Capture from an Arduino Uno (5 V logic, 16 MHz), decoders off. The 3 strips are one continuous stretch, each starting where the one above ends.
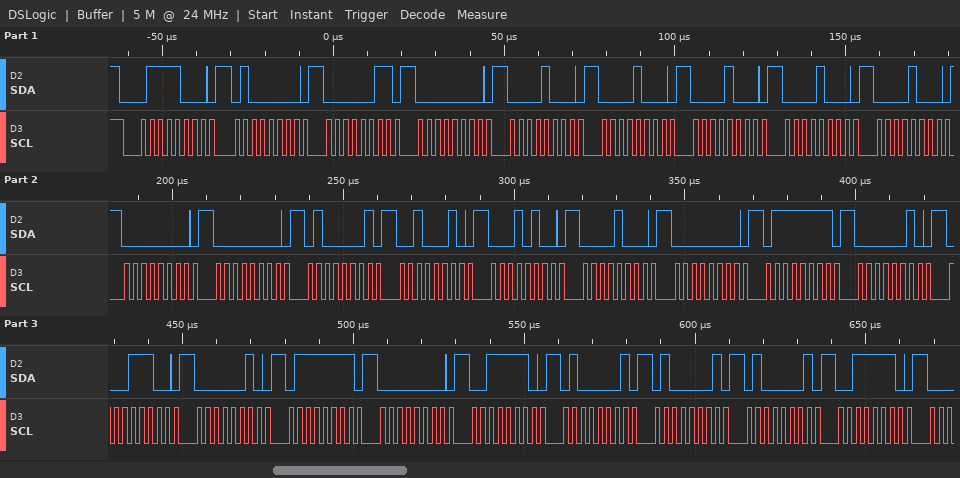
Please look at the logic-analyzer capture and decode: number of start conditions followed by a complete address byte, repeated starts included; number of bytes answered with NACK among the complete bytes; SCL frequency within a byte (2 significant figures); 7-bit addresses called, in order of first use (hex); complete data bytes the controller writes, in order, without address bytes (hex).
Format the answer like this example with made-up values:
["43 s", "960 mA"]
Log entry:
["1", "0", "400 kHz", "0x3C", "40 03 00 08 08 08 08 08 00 00 41 22 14 08 00 7F 02 1C 02 7F 00 3E 41 41 41 3E"]
